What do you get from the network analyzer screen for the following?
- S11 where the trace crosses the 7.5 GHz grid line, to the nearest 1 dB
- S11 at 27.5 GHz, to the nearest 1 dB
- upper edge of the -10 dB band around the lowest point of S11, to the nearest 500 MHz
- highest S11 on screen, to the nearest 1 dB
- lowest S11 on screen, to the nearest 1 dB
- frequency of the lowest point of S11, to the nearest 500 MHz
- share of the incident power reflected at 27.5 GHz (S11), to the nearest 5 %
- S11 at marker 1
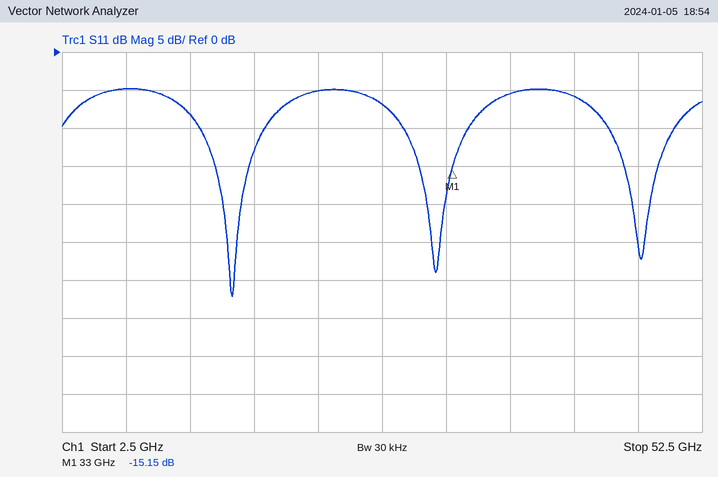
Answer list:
-5 dB
-7 dB
18.5 GHz
-5 dB
-32 dB
16.0 GHz
20 %
-15.15 dB
